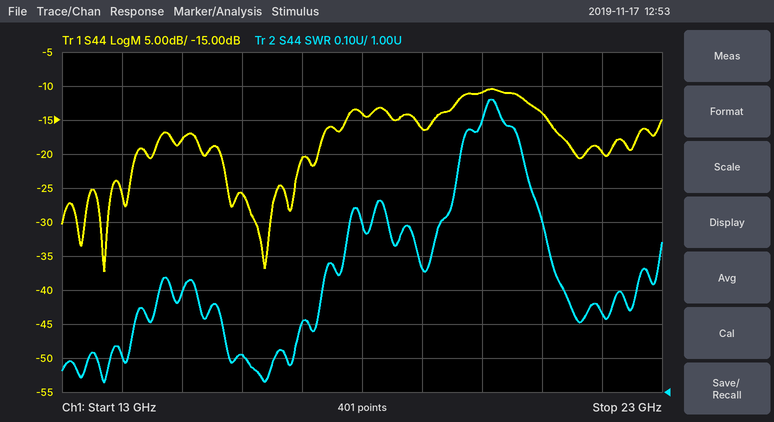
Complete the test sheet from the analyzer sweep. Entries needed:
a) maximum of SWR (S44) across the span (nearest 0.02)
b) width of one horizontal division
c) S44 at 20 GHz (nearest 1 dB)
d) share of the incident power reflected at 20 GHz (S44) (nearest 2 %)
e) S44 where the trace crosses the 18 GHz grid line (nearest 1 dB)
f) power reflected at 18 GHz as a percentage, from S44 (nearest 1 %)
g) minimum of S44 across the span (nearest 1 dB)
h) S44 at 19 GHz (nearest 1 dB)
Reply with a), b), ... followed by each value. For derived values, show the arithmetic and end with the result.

a) 1.86
b) 1 GHz
c) -11 dB
d) 10^(-11/10) ≈ 8 %
e) -14 dB
f) 10^(-14/10) ≈ 4 %
g) -37 dB
h) -16 dB
